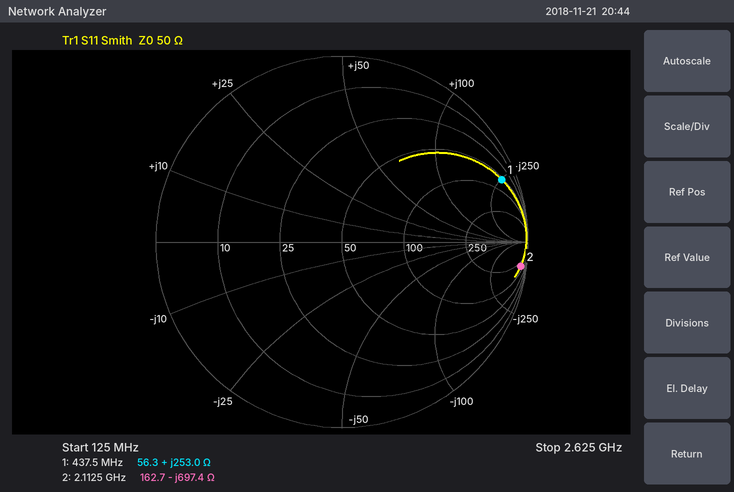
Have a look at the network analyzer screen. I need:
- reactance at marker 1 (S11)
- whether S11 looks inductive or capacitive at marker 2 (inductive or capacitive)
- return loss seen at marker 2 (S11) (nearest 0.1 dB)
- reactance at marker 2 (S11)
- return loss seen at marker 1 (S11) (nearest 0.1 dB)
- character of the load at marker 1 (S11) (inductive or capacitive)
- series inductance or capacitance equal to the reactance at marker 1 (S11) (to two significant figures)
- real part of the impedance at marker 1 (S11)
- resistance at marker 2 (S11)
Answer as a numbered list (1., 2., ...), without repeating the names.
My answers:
1. +253.0 Ω
2. capacitive
3. 0.3 dB
4. -697.4 Ω
5. 0.7 dB
6. inductive
7. 92 nH
8. 56.3 Ω
9. 162.7 Ω
